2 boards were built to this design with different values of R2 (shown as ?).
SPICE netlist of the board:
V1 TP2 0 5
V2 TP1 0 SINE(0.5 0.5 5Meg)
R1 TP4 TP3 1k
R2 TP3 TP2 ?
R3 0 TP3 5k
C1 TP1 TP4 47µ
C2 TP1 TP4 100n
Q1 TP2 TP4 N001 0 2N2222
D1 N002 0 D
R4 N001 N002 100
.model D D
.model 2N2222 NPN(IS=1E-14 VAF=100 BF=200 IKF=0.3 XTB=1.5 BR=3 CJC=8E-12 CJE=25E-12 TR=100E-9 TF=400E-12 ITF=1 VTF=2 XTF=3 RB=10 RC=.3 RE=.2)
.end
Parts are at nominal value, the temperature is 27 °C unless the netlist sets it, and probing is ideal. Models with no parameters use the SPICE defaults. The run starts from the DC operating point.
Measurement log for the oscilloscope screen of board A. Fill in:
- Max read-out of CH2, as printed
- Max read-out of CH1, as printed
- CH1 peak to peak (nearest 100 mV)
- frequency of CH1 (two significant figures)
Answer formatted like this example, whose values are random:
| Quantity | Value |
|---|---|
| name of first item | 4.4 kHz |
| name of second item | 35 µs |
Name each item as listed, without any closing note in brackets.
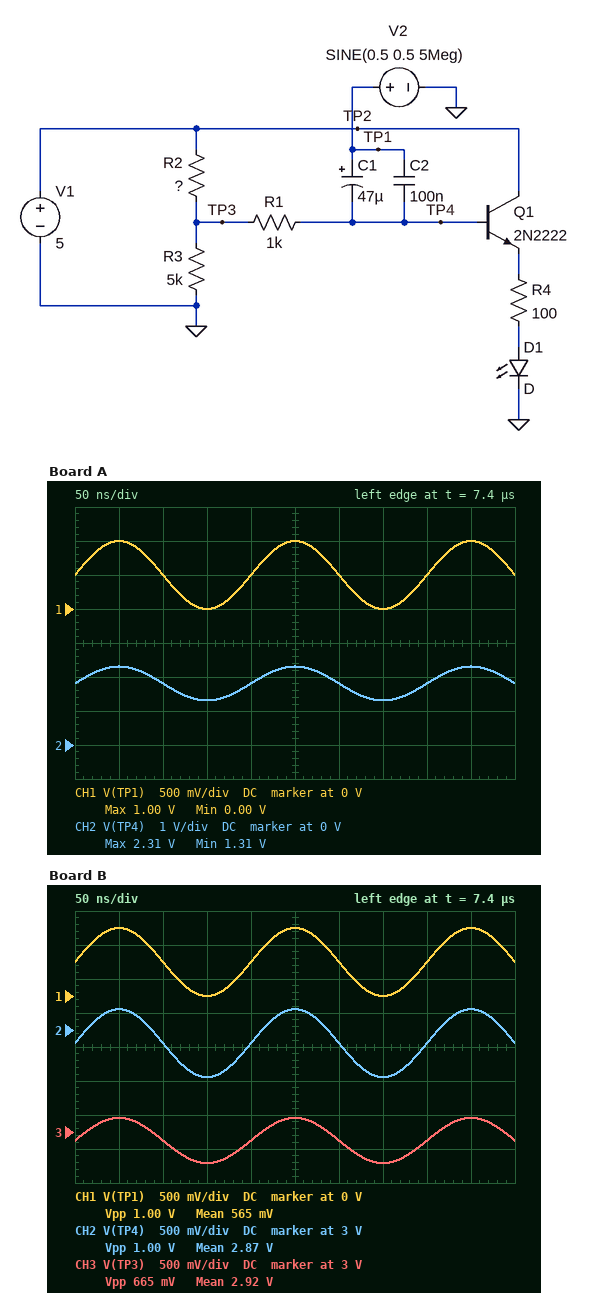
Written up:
| Quantity | Value |
|---|---|
| Max read-out of CH2, as printed | 2.31 V |
| Max read-out of CH1, as printed | 1.00 V |
| CH1 peak to peak | 1.0 V |
| frequency of CH1 | 5.0 MHz |
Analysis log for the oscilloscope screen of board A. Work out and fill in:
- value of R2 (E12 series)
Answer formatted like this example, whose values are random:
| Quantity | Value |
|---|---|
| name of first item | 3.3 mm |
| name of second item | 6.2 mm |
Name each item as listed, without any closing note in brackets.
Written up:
| Quantity | Value |
|---|---|
| value of R2 | 8.2 kΩ |
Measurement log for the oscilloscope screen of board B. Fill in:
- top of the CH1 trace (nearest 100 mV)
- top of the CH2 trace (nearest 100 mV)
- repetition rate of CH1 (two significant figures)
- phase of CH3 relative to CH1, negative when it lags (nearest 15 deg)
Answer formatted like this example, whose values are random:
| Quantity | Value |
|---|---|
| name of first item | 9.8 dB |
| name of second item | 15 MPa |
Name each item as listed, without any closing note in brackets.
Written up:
| Quantity | Value |
|---|---|
| top of the CH1 trace | 1.0 V |
| top of the CH2 trace | 3.3 V |
| repetition rate of CH1 | 5.0 MHz |
| phase of CH3 relative to CH1, negative when it lags | 0 deg |
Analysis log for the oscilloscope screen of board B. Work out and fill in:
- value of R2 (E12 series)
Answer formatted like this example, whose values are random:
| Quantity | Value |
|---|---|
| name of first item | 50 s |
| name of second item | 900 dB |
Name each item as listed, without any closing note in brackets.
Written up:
| Quantity | Value |
|---|---|
| value of R2 | 3.3 kΩ |
